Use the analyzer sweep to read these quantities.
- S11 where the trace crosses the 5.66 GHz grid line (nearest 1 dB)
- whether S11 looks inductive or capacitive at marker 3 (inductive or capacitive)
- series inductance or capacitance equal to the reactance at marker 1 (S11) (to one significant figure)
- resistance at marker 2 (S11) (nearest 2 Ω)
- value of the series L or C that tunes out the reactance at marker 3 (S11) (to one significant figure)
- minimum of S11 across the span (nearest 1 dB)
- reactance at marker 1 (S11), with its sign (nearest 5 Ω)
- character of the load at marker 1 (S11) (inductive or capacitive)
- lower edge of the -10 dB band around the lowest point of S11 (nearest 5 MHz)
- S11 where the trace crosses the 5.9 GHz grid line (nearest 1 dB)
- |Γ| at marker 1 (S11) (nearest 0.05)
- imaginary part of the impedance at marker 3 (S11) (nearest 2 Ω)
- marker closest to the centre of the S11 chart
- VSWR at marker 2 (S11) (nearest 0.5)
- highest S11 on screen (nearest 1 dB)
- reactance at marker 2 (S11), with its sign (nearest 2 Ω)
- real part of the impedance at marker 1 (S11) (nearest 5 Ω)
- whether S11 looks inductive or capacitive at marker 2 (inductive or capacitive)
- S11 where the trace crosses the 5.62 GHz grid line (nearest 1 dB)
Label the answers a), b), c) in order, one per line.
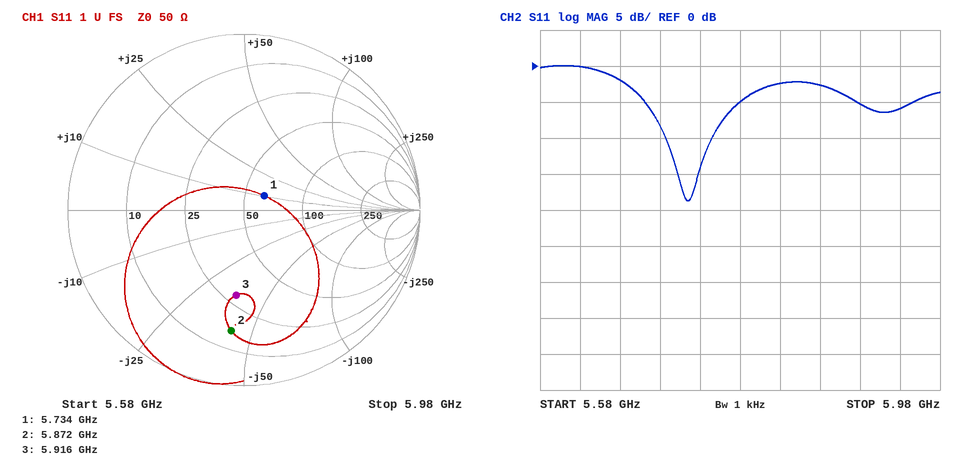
a) -2 dB
b) capacitive
c) 300 pH
d) 16 Ω
e) 1.0 nH
f) -19 dB
g) +10 Ω
h) inductive
i) 5.705 GHz
j) -5 dB
k) 0.15
l) -36 Ω
m) marker 1
n) 5.5
o) 0 dB
p) -42 Ω
q) 60 Ω
r) capacitive
s) 0 dB
